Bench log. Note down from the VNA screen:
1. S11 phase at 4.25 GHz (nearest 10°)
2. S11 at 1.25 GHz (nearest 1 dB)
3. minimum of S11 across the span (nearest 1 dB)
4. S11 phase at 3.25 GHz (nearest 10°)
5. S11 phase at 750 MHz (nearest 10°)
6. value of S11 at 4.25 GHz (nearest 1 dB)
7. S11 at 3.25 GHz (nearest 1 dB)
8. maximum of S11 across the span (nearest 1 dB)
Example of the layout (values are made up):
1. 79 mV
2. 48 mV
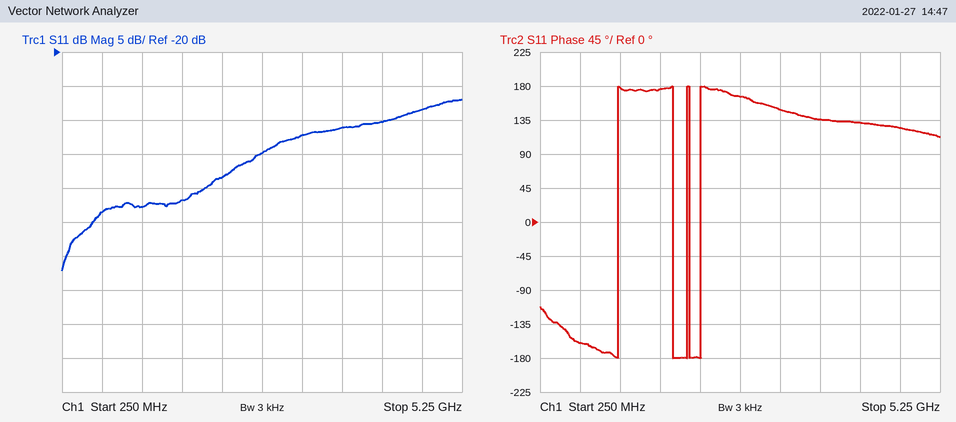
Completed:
1. 130°
2. -43 dB
3. -52 dB
4. 150°
5. -160°
6. -30 dB
7. -32 dB
8. -27 dB
